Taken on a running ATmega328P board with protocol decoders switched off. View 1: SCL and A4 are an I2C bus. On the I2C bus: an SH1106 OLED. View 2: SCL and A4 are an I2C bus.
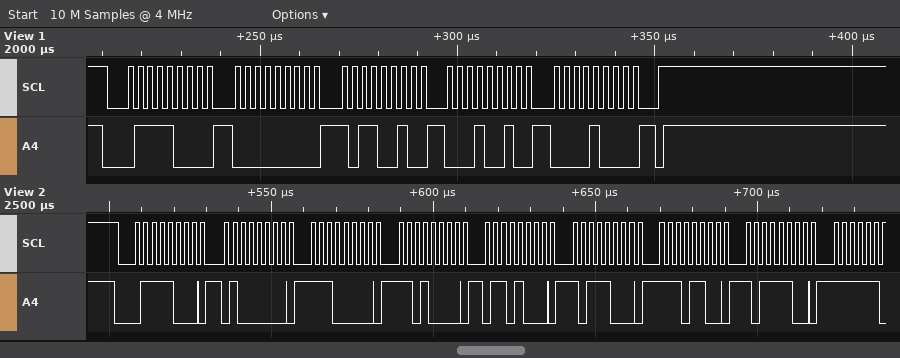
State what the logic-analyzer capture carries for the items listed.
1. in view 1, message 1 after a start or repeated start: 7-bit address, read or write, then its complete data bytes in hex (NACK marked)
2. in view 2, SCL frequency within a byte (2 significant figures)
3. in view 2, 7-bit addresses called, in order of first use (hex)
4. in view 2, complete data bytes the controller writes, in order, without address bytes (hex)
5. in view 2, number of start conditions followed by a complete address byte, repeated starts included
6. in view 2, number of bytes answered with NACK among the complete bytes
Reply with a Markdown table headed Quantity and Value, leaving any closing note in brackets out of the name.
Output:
| Quantity | Value |
|---|---|
| in view 1, message 1 after a start or repeated start: 7-bit address, read or write, then its complete data bytes in hex | 0x3C write: 00 B2 12 08 |
| in view 2, SCL frequency within a byte | 400 kHz |
| in view 2, 7-bit addresses called, in order of first use | 0x3C |
| in view 2, complete data bytes the controller writes, in order, without address bytes | 40 E0 D0 68 B8 EC BC |
| in view 2, number of start conditions followed by a complete address byte, repeated starts included | 1 |
| in view 2, number of bytes answered with NACK among the complete bytes | 0 |
